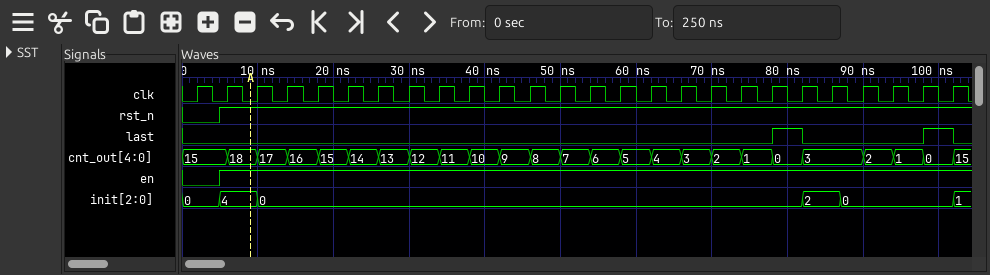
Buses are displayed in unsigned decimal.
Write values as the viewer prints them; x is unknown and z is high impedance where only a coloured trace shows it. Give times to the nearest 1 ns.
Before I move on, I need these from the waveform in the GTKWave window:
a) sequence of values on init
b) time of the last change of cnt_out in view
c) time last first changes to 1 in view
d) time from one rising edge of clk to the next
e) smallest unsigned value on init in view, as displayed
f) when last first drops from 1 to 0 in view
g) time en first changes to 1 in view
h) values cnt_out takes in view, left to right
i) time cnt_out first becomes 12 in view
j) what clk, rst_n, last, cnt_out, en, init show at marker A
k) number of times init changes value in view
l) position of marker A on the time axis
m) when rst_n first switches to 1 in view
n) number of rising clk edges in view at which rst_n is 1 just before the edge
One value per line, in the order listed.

0, 4, 0, 2, 0, 1
102 ns
78 ns
4 ns
0
82 ns
5 ns
15, 18, 17, 16, 15, 14, 13, 12, 11, 10, 9, 8, 7, 6, 5, 4, 3, 2, 1, 0, 3, 2, 1, 0, 15
30 ns
clk=0, rst_n=1, last=0, cnt_out=18, en=1, init=4
5
9 ns
5 ns
25
